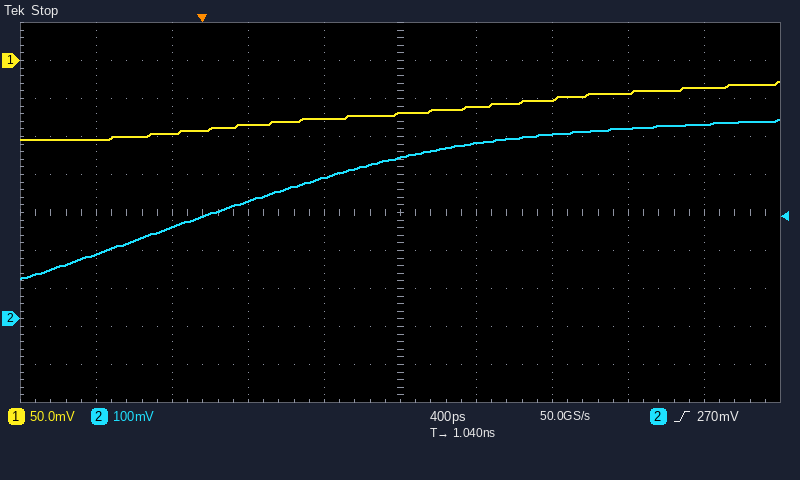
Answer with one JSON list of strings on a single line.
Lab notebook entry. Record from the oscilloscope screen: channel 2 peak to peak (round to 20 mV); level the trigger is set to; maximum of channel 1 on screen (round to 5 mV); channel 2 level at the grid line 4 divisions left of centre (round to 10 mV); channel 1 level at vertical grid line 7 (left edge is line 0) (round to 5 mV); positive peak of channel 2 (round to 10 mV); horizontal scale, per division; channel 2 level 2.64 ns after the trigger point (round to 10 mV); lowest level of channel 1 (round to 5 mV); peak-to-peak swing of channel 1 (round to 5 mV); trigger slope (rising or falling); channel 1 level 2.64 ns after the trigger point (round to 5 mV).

["420 mV", "270 mV", "-30 mV", "170 mV", "-50 mV", "520 mV", "400 ps", "510 mV", "-105 mV", "75 mV", "rising", "-35 mV"]
